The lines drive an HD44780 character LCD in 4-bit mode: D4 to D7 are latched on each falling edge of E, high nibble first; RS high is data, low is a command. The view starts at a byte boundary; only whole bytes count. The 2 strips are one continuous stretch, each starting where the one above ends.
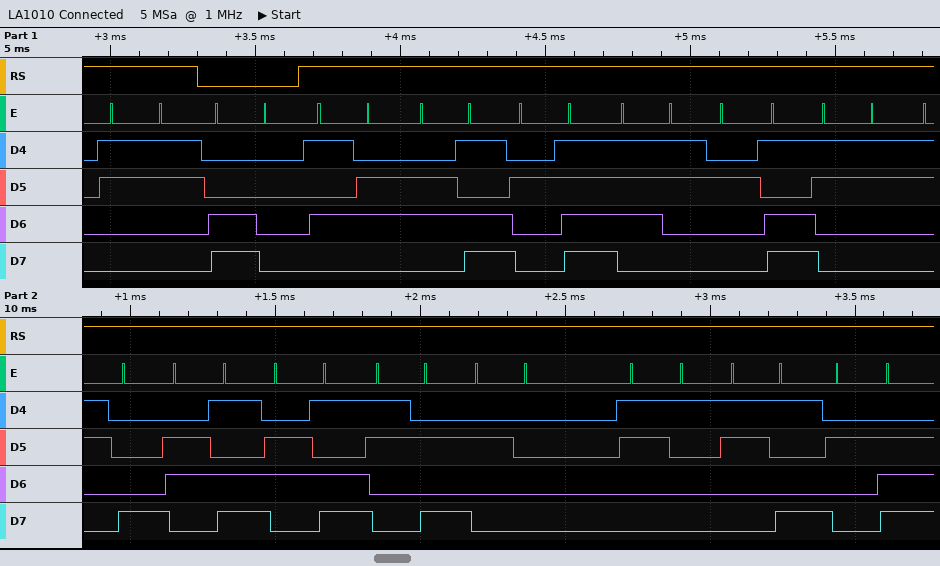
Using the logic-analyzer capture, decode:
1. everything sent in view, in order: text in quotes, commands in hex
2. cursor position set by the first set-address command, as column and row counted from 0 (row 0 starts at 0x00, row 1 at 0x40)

"3" 0xC0 "Vm/s-38mm: 19."
column 0, row 1
